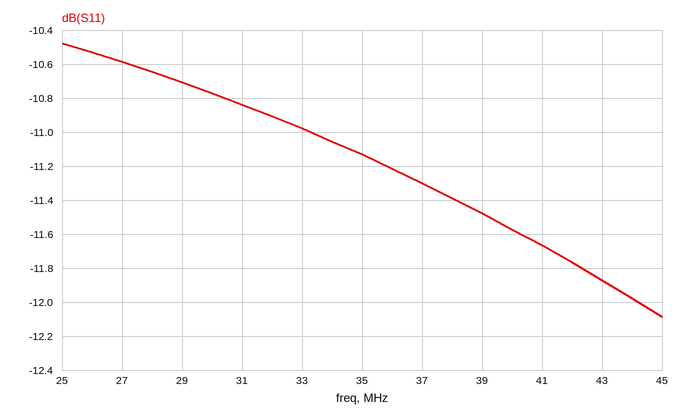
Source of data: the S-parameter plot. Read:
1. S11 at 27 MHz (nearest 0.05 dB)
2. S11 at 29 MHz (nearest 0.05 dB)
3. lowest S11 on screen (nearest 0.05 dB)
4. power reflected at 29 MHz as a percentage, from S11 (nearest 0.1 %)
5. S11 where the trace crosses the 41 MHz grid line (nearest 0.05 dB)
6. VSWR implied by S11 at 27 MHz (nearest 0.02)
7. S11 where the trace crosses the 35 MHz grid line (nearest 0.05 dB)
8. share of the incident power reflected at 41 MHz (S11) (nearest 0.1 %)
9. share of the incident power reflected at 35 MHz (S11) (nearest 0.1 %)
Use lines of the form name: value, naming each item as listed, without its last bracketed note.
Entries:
S11 at 27 MHz: -10.60 dB
S11 at 29 MHz: -10.70 dB
lowest S11 on screen: -12.10 dB
power reflected at 29 MHz as a percentage, from S11: 8.5 %
S11 where the trace crosses the 41 MHz grid line: -11.65 dB
VSWR implied by S11 at 27 MHz: 1.84
S11 where the trace crosses the 35 MHz grid line: -11.15 dB
share of the incident power reflected at 41 MHz (S11): 6.8 %
share of the incident power reflected at 35 MHz (S11): 7.7 %
